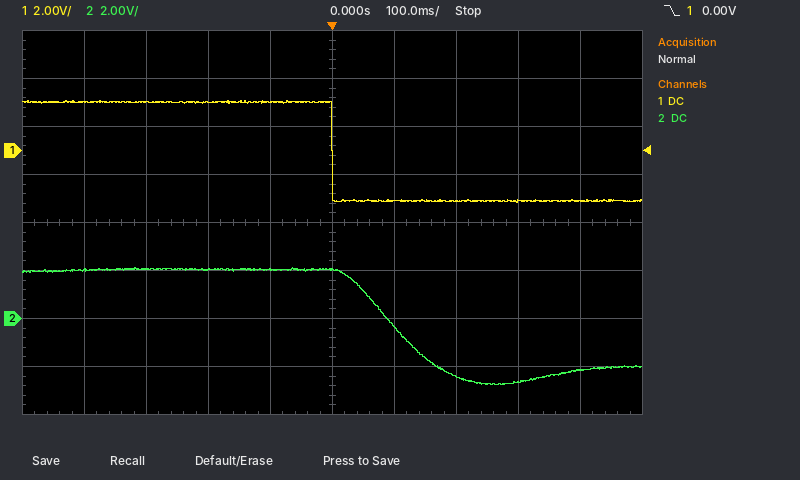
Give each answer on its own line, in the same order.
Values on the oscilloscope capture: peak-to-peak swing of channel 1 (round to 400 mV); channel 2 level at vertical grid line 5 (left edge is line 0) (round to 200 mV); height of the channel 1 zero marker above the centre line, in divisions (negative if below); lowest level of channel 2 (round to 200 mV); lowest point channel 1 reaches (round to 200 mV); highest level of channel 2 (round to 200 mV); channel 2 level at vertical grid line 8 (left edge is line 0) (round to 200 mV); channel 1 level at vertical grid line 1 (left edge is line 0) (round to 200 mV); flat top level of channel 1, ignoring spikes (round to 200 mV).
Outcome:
4.4 V
2.0 V
+1.5 div
-2.8 V
-2.2 V
2.2 V
-2.6 V
2.0 V
2.0 V
